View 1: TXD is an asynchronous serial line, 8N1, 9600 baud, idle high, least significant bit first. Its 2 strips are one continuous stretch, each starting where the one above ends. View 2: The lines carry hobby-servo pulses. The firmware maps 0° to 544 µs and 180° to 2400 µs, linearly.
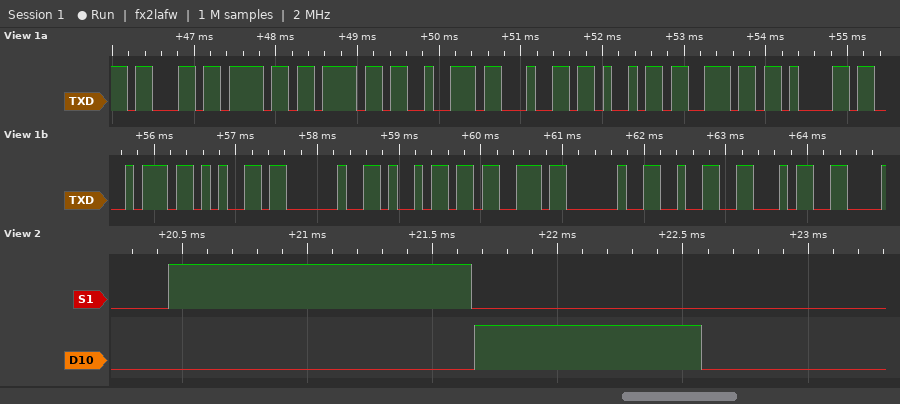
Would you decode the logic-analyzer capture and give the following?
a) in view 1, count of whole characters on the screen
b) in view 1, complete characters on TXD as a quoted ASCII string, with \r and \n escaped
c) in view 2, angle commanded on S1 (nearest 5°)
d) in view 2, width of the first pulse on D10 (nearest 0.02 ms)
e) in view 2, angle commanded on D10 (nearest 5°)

16
"coordinate is 24"
65°
0.90 ms
35°
